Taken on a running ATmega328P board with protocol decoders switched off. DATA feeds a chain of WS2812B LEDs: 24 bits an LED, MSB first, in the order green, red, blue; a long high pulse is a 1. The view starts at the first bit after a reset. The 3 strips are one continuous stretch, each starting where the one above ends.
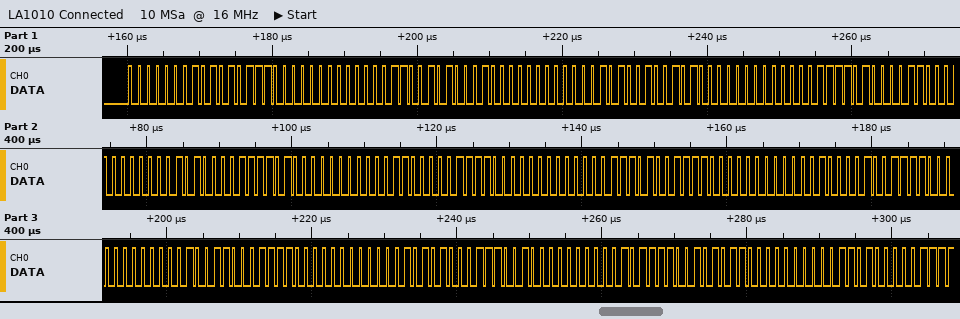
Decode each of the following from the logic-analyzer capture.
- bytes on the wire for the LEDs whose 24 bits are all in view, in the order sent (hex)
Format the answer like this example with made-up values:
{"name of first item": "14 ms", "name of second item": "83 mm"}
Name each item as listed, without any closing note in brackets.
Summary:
{"bytes on the wire for the LEDs whose 24 bits are all in view, in the order sent": "01 57 00 06 51 00 0A 4A 00 0F 43 00 14 3D 00 18 3C 00 1D 3C 00 21 3C 00 26 3C 00 2A 39 00 2F 2B 00"}
